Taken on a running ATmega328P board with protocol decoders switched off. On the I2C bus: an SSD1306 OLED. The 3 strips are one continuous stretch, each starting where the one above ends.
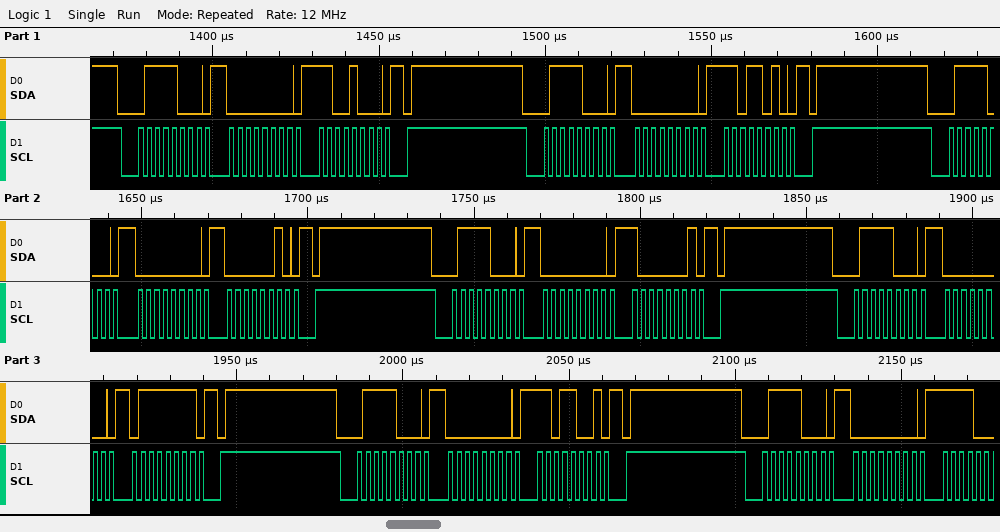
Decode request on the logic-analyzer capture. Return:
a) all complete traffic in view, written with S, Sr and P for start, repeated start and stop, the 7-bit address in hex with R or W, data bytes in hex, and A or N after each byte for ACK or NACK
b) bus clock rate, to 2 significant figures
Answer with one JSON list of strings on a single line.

["S 3CW A 00 A C8 A P S 3CW A 00 A DA A P S 3CW A 00 A 02 A P S 3CW A 00 A 81 A P S 3CW A 00 A 7F A P S 3CW A 00 A D9 A P S 3CW A 00 A", "400 kHz"]
